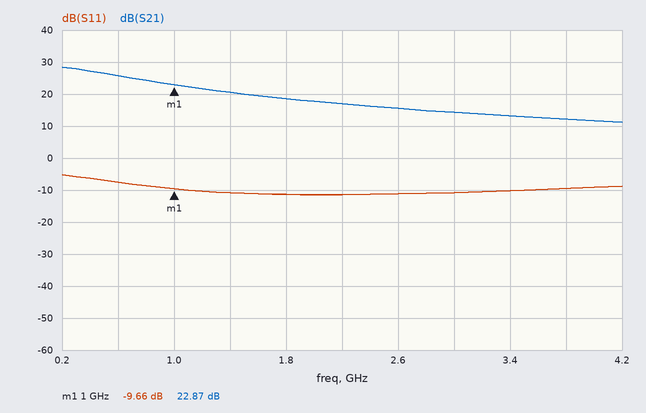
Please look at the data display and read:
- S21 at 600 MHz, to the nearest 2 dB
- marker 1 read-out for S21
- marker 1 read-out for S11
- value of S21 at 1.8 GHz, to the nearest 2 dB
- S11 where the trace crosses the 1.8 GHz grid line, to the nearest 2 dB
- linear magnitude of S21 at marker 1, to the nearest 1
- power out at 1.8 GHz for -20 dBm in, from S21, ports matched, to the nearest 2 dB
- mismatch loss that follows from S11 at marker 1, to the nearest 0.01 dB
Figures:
26 dB
22.87 dB
-9.66 dB
18 dB
-12 dB
14
-2 dBm
0.50 dB
